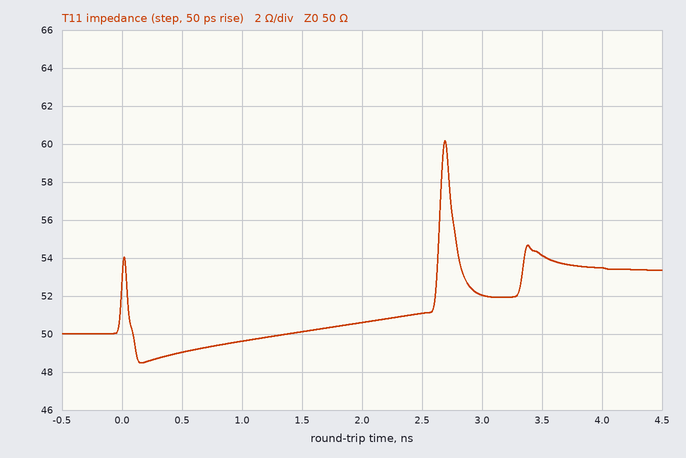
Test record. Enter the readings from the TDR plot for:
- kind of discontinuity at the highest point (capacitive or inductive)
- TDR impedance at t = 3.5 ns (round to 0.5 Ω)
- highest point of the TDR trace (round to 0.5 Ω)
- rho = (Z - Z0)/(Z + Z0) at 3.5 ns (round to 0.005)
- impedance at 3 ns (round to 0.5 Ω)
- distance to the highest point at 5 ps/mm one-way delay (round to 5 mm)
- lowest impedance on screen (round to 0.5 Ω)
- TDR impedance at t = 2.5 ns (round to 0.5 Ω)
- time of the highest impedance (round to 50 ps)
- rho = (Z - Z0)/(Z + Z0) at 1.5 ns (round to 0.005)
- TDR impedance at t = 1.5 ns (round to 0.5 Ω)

inductive
54.0 Ω
60.0 Ω
+0.040
52.0 Ω
270 mm
48.5 Ω
51.0 Ω
2.70 ns
0.000
50.0 Ω
